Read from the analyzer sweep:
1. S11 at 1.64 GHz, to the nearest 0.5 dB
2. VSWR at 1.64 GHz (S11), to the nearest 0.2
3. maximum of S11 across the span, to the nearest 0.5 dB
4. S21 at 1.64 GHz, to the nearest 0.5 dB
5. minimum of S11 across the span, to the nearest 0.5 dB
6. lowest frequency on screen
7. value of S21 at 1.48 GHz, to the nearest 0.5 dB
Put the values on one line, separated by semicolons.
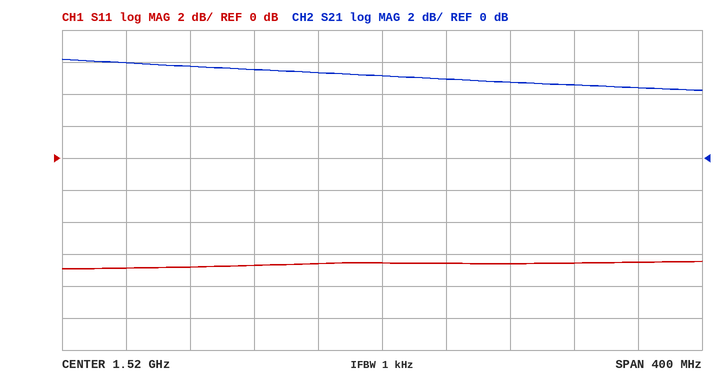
-6.5 dB; 2.8; -6.5 dB; 4.5 dB; -7.0 dB; 1.32 GHz; 5.5 dB
